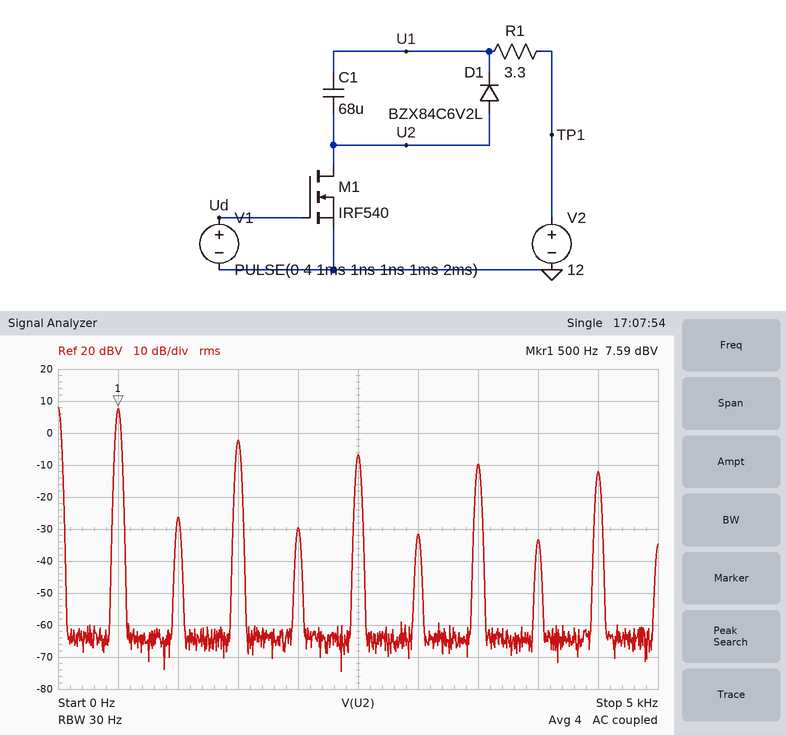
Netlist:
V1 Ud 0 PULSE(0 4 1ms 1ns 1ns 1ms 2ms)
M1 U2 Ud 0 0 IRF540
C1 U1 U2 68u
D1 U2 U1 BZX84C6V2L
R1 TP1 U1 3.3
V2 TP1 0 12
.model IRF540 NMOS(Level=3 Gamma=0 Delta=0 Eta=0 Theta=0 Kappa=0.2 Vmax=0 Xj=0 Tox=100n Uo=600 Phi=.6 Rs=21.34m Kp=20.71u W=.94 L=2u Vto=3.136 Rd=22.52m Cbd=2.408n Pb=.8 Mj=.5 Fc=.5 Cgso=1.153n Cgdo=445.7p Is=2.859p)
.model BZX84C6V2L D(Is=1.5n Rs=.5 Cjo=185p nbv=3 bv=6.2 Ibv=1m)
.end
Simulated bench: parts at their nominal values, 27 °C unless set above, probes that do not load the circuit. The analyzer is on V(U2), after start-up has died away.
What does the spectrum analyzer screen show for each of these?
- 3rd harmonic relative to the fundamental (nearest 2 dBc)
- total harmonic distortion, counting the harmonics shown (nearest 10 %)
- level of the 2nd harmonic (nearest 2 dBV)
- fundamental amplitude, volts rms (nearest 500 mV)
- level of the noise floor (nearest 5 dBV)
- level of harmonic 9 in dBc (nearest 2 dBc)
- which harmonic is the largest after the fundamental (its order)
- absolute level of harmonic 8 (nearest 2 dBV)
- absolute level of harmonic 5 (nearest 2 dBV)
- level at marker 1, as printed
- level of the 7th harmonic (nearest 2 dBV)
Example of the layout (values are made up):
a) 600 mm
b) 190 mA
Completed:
a) -10 dBc
b) 40 %
c) -26 dBV
d) 2.5 V
e) -65 dBV
f) -20 dBc
g) 3
h) -34 dBV
i) -6 dBV
j) 7.59 dBV
k) -10 dBV
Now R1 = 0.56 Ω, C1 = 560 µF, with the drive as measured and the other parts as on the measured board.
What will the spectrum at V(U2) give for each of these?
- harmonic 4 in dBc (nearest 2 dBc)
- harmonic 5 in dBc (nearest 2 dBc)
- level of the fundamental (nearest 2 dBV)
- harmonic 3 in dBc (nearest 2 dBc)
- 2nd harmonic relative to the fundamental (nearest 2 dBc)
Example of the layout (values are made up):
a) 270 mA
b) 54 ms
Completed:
a) -58 dBc
b) -18 dBc
c) 2 dBV
d) -12 dBc
e) -44 dBc
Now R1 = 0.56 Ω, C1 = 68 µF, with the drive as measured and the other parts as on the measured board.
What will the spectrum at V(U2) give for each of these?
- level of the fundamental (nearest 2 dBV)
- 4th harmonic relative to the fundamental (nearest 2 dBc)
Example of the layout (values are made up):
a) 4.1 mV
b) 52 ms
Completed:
a) 4 dBV
b) -38 dBc
